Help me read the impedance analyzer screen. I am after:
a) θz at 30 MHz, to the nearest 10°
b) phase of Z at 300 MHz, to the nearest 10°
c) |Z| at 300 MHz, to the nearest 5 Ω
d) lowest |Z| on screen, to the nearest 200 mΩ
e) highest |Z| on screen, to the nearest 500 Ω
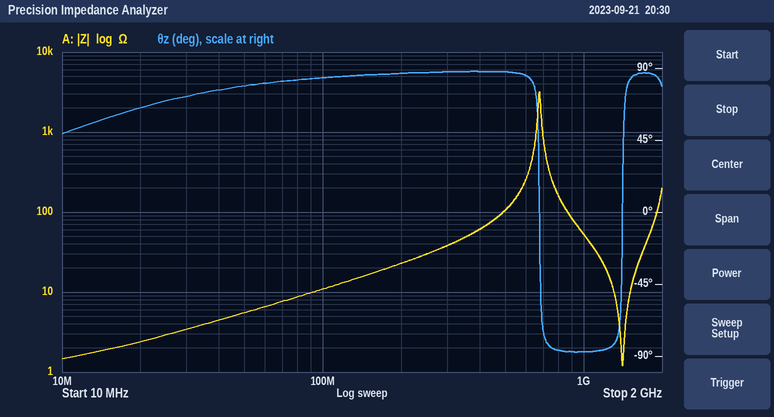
70°
90°
40 Ω
1.2 Ω
3.0 kΩ
